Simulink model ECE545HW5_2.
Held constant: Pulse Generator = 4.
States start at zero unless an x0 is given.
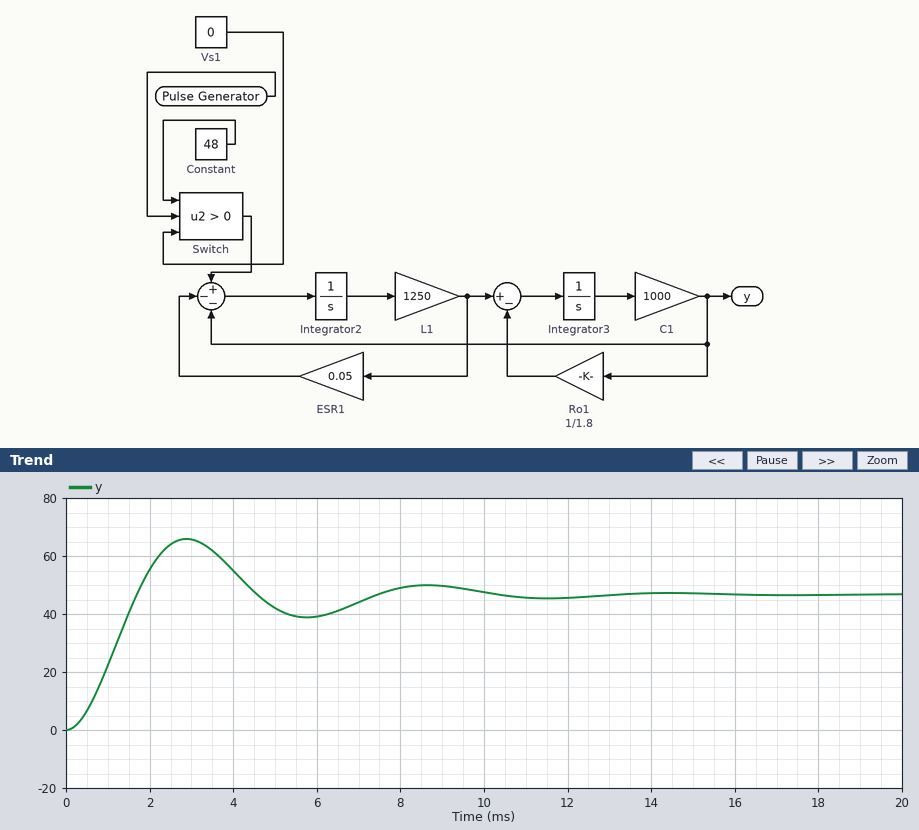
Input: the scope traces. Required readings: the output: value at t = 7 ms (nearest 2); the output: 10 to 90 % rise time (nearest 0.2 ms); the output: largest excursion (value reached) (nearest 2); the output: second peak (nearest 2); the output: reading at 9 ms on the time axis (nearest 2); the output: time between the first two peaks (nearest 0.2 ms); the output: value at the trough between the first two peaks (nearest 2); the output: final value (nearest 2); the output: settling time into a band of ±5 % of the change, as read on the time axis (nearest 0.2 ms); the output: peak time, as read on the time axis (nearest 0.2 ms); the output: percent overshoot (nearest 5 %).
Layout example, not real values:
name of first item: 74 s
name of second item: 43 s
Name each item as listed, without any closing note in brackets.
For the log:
the output: value at t = 7 ms: 44
the output: 10 to 90 % rise time: 1.2 ms
the output: largest excursion (value reached): 66
the output: second peak: 50
the output: reading at 9 ms on the time axis: 50
the output: time between the first two peaks: 5.8 ms
the output: value at the trough between the first two peaks: 38
the output: final value: 46
the output: settling time into a band of ±5 % of the change, as read on the time axis: 9.4 ms
the output: peak time, as read on the time axis: 2.8 ms
the output: percent overshoot: 40 %
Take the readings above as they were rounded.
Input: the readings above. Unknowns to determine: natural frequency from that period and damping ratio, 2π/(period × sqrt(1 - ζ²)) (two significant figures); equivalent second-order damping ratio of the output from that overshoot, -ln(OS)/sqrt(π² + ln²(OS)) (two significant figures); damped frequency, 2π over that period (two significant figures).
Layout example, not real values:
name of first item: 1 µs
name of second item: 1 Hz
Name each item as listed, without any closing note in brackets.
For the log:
natural frequency from that period and damping ratio, 2π/(period × sqrt(1 - ζ²)): 1.1 rad/ms
equivalent second-order damping ratio of the output from that overshoot, -ln(OS)/sqrt(π² + ln²(OS)): 0.28
damped frequency, 2π over that period: 1.1 rad/ms
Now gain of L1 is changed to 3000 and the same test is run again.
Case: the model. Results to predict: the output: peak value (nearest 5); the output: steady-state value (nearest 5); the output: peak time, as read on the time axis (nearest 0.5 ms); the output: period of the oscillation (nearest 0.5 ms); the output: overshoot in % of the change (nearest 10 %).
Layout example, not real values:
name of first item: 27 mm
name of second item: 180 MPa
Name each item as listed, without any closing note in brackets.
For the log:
the output: peak value: 70
the output: steady-state value: 45
the output: peak time, as read on the time axis: 2.0 ms
the output: period of the oscillation: 3.5 ms
the output: overshoot in % of the change: 50 %
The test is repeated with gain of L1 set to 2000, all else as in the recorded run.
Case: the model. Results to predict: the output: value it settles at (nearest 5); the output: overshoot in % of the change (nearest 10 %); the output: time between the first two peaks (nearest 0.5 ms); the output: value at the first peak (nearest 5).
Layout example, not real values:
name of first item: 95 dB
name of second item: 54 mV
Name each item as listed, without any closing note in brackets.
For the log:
the output: value it settles at: 45
the output: overshoot in % of the change: 50 %
the output: time between the first two peaks: 4.5 ms
the output: value at the first peak: 70
